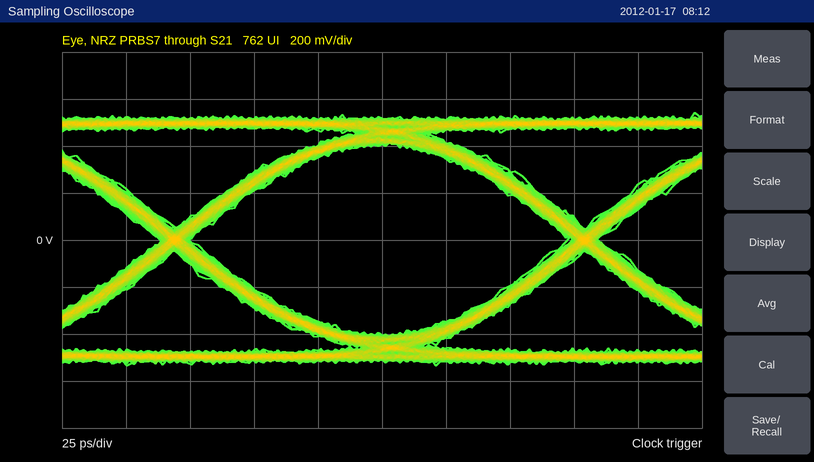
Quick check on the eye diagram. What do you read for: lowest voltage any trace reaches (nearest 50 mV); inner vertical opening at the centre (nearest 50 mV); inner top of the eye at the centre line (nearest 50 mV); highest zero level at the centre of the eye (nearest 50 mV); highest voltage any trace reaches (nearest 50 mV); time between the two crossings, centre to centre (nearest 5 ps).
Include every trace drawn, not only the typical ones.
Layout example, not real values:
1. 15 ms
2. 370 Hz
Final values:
1. -550 mV
2. 800 mV
3. 400 mV
4. -400 mV
5. 550 mV
6. 160 ps
